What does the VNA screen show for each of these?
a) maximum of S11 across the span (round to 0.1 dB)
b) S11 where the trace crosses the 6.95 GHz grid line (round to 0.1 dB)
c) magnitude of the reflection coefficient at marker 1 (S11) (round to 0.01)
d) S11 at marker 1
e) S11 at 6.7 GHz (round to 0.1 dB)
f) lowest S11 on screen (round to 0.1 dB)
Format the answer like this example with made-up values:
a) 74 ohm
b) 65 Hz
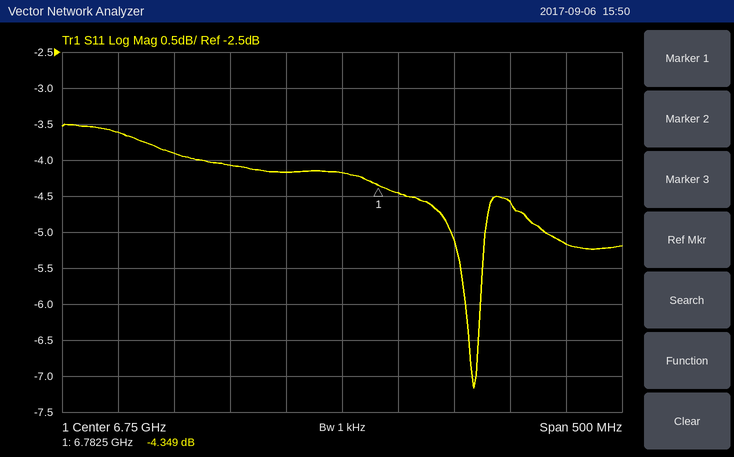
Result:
a) -3.5 dB
b) -5.2 dB
c) 0.61
d) -4.349 dB
e) -4.2 dB
f) -7.2 dB
